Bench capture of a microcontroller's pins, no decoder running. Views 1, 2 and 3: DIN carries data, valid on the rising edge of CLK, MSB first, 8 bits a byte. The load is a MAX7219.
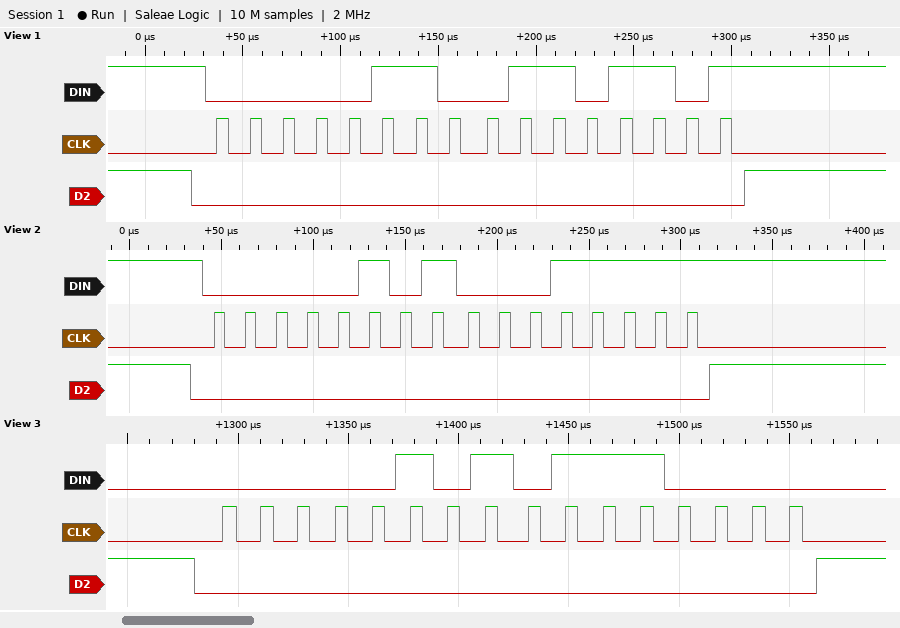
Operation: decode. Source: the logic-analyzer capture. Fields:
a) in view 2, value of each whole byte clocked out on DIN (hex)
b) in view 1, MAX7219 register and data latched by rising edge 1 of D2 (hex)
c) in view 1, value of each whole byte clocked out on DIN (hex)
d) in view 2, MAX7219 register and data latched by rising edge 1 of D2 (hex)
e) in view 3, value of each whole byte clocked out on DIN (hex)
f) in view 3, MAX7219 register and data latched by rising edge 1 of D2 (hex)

05 1F
register 0x6, data 0x6D
06 6D
register 0x5, data 0x1F
05 70
register 0x5, data 0x70
